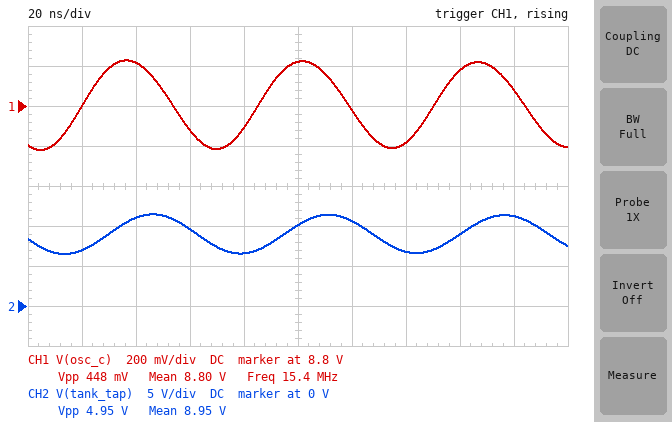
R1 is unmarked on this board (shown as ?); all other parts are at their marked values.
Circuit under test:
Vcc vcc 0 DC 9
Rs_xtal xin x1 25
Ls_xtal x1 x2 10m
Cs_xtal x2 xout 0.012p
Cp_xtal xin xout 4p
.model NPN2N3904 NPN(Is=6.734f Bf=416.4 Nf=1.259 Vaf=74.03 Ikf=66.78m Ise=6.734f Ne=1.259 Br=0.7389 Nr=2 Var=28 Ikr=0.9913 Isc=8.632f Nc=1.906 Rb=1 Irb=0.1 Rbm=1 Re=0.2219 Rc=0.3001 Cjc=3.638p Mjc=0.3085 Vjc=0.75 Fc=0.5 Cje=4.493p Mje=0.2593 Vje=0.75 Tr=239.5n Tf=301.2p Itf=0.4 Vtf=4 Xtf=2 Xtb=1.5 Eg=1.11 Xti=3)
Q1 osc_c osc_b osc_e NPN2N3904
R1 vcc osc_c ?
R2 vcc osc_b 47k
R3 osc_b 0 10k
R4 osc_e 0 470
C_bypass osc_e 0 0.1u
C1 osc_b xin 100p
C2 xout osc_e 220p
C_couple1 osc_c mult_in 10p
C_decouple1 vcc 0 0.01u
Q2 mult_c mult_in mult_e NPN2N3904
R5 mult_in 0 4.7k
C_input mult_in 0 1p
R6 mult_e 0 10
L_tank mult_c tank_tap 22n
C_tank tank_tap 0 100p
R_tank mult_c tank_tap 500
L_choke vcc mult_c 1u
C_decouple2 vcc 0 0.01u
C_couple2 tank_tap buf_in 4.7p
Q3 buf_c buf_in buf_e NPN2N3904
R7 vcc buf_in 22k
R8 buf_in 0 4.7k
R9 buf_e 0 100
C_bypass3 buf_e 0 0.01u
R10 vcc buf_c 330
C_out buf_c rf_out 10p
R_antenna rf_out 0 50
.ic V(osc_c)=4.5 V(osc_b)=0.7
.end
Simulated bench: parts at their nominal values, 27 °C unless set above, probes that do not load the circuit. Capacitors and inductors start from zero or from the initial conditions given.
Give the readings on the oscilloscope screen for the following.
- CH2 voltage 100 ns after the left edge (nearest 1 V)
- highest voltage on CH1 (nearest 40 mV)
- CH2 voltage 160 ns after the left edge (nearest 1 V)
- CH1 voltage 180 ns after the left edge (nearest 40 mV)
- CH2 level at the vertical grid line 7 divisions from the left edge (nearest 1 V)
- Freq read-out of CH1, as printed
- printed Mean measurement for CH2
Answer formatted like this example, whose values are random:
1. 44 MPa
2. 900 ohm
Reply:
1. 10 V
2. 9.04 V
3. 9 V
4. 8.88 V
5. 7 V
6. 15.4 MHz
7. 8.95 V
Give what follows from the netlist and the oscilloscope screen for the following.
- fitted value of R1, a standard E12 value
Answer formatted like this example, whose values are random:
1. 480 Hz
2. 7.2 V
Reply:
1. 1.8 kΩ
